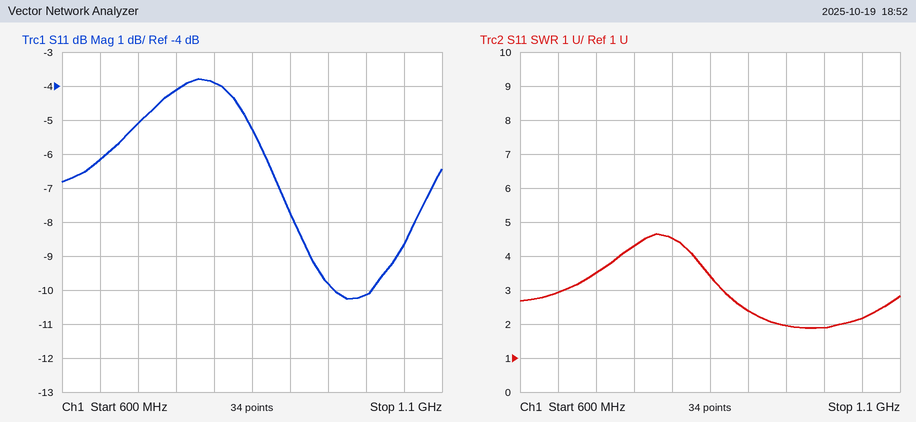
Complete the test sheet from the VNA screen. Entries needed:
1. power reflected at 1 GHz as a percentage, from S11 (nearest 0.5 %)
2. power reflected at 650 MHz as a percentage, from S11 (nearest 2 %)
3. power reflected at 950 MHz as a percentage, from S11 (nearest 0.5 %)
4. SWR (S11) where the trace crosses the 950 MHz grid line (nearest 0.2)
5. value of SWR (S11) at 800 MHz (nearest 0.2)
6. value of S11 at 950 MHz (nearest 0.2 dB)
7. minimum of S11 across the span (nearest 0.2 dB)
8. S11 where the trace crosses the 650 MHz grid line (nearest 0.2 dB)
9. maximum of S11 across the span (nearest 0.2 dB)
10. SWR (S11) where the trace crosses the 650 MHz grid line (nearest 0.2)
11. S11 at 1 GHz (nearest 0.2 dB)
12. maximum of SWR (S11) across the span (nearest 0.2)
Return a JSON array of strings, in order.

["9.5 %", "24 %", "10.5 %", "2.0", "4.6", "-9.8 dB", "-10.2 dB", "-6.2 dB", "-3.8 dB", "3.0", "-10.2 dB", "4.6"]
